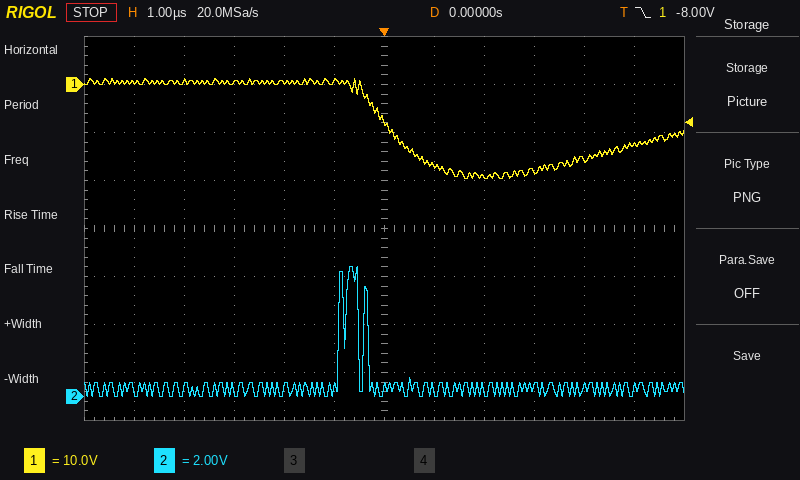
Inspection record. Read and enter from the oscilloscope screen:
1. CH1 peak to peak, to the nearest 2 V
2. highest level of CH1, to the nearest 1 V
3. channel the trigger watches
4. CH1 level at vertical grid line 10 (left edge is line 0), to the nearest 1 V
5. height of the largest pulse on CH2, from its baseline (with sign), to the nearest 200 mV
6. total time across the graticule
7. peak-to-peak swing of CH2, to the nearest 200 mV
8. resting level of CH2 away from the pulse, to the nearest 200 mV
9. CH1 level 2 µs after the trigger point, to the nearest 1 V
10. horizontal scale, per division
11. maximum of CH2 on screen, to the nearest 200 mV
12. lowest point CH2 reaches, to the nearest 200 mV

20 V
1 V
CH1
-16 V
+5.0 V
12 µs
5.4 V
400 mV
-19 V
1 µs
5.4 V
0.0 V
